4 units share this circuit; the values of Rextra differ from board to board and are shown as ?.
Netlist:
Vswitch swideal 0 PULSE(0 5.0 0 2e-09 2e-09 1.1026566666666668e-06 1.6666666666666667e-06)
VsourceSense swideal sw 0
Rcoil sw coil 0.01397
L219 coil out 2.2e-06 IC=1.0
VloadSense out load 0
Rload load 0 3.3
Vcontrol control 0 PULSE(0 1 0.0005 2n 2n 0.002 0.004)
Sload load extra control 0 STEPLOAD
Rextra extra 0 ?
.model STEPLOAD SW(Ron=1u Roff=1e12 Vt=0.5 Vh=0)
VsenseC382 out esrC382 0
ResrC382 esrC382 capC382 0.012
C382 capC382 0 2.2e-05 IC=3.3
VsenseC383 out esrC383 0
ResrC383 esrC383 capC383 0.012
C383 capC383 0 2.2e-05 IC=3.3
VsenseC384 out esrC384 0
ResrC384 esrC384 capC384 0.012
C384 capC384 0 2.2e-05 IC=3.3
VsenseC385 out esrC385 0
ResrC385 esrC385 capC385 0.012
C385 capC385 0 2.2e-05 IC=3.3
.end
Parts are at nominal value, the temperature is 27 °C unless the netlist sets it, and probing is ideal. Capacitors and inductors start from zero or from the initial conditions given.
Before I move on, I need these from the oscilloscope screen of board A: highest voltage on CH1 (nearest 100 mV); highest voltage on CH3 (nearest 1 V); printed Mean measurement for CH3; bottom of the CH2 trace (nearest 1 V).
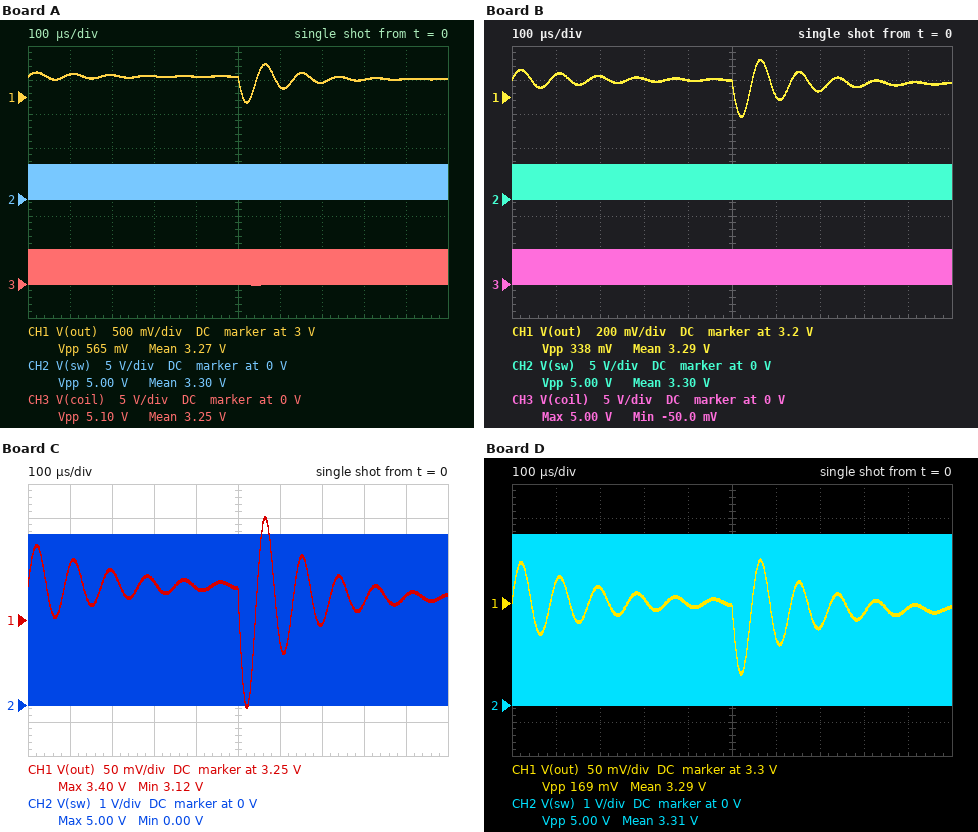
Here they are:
3.5 V
5 V
3.25 V
0 V
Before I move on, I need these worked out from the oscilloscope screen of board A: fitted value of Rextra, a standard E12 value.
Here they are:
1.2 Ω
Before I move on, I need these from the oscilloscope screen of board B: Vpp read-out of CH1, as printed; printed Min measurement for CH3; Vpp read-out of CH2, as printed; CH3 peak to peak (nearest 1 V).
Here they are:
338 mV
-50.0 mV
5.00 V
5 V
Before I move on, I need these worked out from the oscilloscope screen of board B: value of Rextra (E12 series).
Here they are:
2.2 Ω
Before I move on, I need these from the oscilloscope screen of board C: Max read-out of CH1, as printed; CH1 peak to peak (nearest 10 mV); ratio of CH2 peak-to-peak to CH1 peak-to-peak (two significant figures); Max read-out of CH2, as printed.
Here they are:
3.40 V
280 mV
18
5.00 V
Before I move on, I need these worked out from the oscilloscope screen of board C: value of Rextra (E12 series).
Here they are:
2.7 Ω
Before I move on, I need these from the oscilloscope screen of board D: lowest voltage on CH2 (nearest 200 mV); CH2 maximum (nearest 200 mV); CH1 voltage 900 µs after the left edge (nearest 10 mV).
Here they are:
0 V
5.0 V
3.29 V
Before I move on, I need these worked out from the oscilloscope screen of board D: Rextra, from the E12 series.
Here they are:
4.7 Ω
